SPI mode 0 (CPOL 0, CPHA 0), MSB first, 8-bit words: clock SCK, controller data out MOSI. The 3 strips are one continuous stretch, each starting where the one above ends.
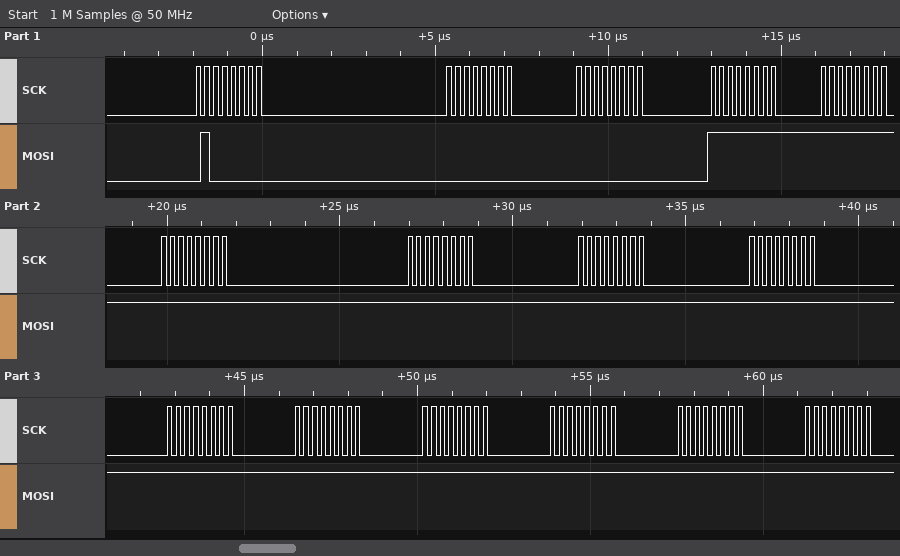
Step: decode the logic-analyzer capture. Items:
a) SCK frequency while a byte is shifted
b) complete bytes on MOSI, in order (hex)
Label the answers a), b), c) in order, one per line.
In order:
a) 4 MHz
b) 40 00 00 FF FF FF FF FF FF FF FF FF FF FF FF
